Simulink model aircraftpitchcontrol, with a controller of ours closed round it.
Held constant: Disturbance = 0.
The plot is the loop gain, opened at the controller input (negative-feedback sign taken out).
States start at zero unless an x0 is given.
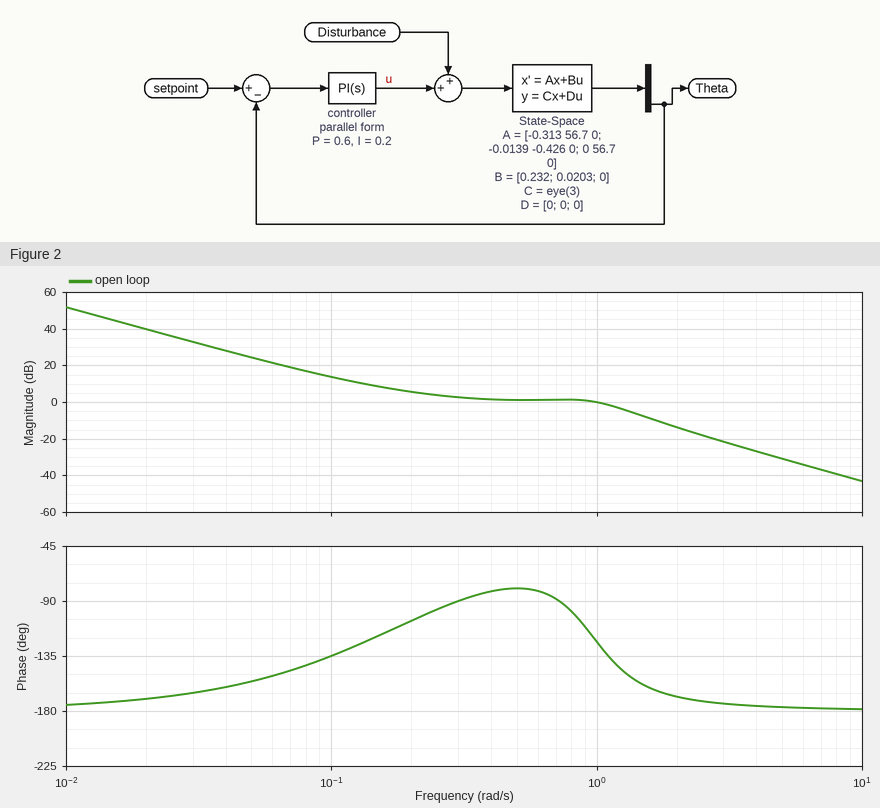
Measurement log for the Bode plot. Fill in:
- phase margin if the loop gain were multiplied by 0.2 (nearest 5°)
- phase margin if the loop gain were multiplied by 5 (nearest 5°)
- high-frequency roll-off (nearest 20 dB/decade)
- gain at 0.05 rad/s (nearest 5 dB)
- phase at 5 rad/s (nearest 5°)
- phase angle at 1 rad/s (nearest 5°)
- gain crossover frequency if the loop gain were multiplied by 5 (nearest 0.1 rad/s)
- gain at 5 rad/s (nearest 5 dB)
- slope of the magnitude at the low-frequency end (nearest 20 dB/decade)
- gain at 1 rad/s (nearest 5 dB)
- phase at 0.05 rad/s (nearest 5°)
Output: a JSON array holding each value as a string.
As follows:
["45°", "10°", "-40 dB/decade", "25 dB", "-175°", "-125°", "2.0 rad/s", "-30 dB", "-40 dB/decade", "0 dB", "-155°"]
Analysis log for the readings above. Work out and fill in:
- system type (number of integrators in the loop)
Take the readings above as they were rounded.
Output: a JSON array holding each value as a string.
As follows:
["2"]
